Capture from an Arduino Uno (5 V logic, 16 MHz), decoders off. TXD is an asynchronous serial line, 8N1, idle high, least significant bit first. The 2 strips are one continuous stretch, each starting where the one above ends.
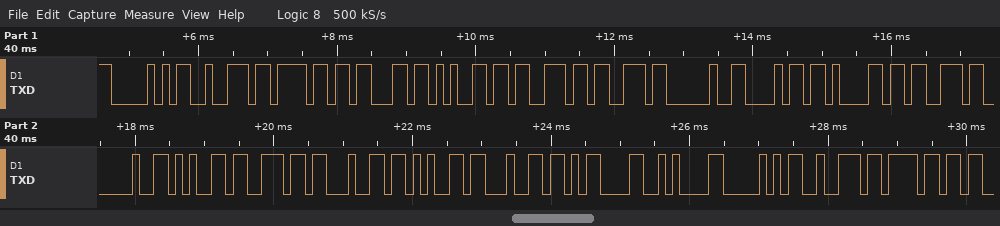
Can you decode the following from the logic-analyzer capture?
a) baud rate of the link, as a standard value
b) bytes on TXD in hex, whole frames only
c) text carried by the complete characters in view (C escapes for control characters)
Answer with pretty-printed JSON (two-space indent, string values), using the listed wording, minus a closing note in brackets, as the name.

{
  "baud rate of the link, as a standard value": "9600 baud",
  "bytes on TXD in hex, whole frames only": "50 72 6F 63 65 73 73 20 68 61 73 20 65 6E 64 65 64 0D 0A 50 72 6F",
  "text carried by the complete characters in view": "\"Process has ended\\r\\nPro\""
}
